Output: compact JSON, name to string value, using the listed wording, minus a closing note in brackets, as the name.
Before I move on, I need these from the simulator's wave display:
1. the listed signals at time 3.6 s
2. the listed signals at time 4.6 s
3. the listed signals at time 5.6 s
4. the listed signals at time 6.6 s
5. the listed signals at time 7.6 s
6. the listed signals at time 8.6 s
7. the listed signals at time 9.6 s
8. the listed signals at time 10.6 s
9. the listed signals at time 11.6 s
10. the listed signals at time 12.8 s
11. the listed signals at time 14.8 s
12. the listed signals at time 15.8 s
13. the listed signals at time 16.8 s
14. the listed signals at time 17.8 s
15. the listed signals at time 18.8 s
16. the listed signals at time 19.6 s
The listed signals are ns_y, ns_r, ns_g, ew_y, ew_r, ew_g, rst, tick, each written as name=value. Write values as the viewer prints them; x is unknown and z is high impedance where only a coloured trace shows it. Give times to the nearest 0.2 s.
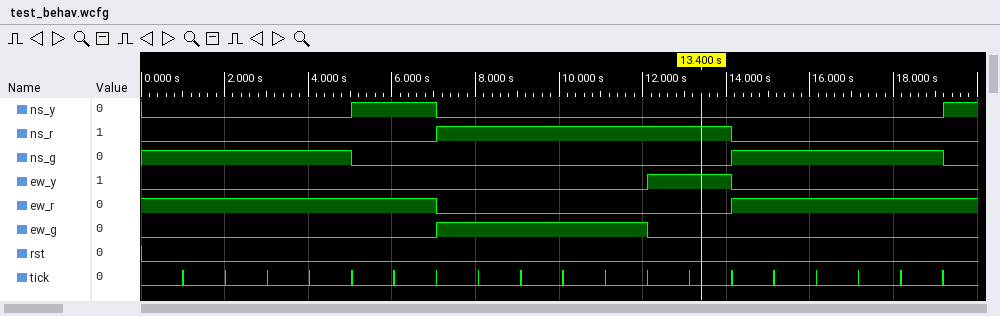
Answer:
{"the listed signals at time 3.6 s": "ns_y=0, ns_r=0, ns_g=1, ew_y=0, ew_r=1, ew_g=0, rst=0, tick=0", "the listed signals at time 4.6 s": "ns_y=0, ns_r=0, ns_g=1, ew_y=0, ew_r=1, ew_g=0, rst=0, tick=0", "the listed signals at time 5.6 s": "ns_y=1, ns_r=0, ns_g=0, ew_y=0, ew_r=1, ew_g=0, rst=0, tick=0", "the listed signals at time 6.6 s": "ns_y=1, ns_r=0, ns_g=0, ew_y=0, ew_r=1, ew_g=0, rst=0, tick=0", "the listed signals at time 7.6 s": "ns_y=0, ns_r=1, ns_g=0, ew_y=0, ew_r=0, ew_g=1, rst=0, tick=0", "the listed signals at time 8.6 s": "ns_y=0, ns_r=1, ns_g=0, ew_y=0, ew_r=0, ew_g=1, rst=0, tick=0", "the listed signals at time 9.6 s": "ns_y=0, ns_r=1, ns_g=0, ew_y=0, ew_r=0, ew_g=1, rst=0, tick=0", "the listed signals at time 10.6 s": "ns_y=0, ns_r=1, ns_g=0, ew_y=0, ew_r=0, ew_g=1, rst=0, tick=0", "the listed signals at time 11.6 s": "ns_y=0, ns_r=1, ns_g=0, ew_y=0, ew_r=0, ew_g=1, rst=0, tick=0", "the listed signals at time 12.8 s": "ns_y=0, ns_r=1, ns_g=0, ew_y=1, ew_r=0, ew_g=0, rst=0, tick=0", "the listed signals at time 14.8 s": "ns_y=0, ns_r=0, ns_g=1, ew_y=0, ew_r=1, ew_g=0, rst=0, tick=0", "the listed signals at time 15.8 s": "ns_y=0, ns_r=0, ns_g=1, ew_y=0, ew_r=1, ew_g=0, rst=0, tick=0", "the listed signals at time 16.8 s": "ns_y=0, ns_r=0, ns_g=1, ew_y=0, ew_r=1, ew_g=0, rst=0, tick=0", "the listed signals at time 17.8 s": "ns_y=0, ns_r=0, ns_g=1, ew_y=0, ew_r=1, ew_g=0, rst=0, tick=0", "the listed signals at time 18.8 s": "ns_y=0, ns_r=0, ns_g=1, ew_y=0, ew_r=1, ew_g=0, rst=0, tick=0", "the listed signals at time 19.6 s": "ns_y=1, ns_r=0, ns_g=0, ew_y=0, ew_r=1, ew_g=0, rst=0, tick=0"}
